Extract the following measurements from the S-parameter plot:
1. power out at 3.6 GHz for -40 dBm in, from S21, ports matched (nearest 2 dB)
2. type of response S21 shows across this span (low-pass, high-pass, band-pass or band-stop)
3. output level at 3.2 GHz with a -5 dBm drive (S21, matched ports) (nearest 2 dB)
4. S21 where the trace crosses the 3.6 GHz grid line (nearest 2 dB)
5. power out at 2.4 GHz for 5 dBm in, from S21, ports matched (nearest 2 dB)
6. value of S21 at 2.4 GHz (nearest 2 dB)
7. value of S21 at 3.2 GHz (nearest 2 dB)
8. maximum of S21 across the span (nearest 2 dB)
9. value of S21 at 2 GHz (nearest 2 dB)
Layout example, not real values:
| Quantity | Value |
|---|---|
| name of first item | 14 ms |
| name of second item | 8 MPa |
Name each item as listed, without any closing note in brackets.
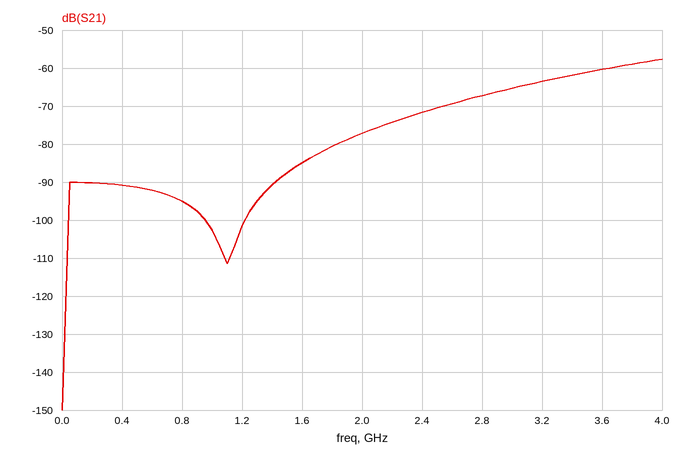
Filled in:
| Quantity | Value |
|---|---|
| power out at 3.6 GHz for -40 dBm in, from S21, ports matched | -100 dBm |
| type of response S21 shows across this span | high-pass |
| output level at 3.2 GHz with a -5 dBm drive (S21, matched ports) | -68 dBm |
| S21 where the trace crosses the 3.6 GHz grid line | -60 dB |
| power out at 2.4 GHz for 5 dBm in, from S21, ports matched | -66 dBm |
| value of S21 at 2.4 GHz | -72 dB |
| value of S21 at 3.2 GHz | -64 dB |
| maximum of S21 across the span | -58 dB |
| value of S21 at 2 GHz | -78 dB |
